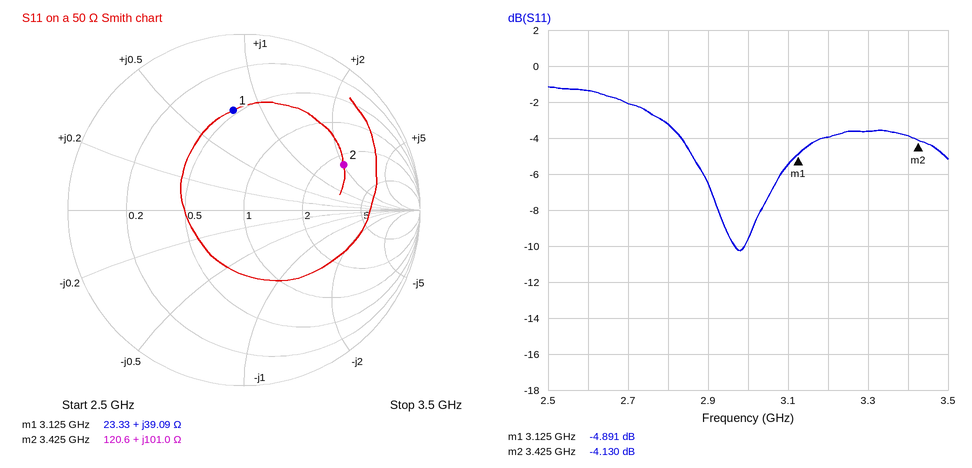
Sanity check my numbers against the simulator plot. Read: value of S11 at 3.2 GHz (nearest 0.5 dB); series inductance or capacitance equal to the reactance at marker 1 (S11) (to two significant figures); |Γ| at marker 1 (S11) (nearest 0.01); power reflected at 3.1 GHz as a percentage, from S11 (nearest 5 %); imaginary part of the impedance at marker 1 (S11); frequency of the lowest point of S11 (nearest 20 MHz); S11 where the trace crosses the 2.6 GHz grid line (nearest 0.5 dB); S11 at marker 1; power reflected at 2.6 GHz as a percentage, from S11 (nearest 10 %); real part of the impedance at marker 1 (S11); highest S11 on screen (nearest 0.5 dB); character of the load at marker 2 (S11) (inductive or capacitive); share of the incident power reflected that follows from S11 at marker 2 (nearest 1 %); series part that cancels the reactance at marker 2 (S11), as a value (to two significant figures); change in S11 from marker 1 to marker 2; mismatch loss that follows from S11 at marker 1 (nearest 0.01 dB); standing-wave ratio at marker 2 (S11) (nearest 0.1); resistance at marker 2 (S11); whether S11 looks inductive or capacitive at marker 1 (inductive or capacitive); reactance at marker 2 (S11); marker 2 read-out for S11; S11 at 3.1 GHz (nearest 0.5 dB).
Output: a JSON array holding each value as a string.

["-4.0 dB", "2.0 nH", "0.57", "30 %", "+39.09 Ω", "2.98 GHz", "-1.5 dB", "-4.891 dB", "70 %", "23.33 Ω", "-1.0 dB", "inductive", "39 %", "460 fF", "0.761 dB", "1.70 dB", "4.3", "120.6 Ω", "inductive", "+101.0 Ω", "-4.130 dB", "-5.5 dB"]
